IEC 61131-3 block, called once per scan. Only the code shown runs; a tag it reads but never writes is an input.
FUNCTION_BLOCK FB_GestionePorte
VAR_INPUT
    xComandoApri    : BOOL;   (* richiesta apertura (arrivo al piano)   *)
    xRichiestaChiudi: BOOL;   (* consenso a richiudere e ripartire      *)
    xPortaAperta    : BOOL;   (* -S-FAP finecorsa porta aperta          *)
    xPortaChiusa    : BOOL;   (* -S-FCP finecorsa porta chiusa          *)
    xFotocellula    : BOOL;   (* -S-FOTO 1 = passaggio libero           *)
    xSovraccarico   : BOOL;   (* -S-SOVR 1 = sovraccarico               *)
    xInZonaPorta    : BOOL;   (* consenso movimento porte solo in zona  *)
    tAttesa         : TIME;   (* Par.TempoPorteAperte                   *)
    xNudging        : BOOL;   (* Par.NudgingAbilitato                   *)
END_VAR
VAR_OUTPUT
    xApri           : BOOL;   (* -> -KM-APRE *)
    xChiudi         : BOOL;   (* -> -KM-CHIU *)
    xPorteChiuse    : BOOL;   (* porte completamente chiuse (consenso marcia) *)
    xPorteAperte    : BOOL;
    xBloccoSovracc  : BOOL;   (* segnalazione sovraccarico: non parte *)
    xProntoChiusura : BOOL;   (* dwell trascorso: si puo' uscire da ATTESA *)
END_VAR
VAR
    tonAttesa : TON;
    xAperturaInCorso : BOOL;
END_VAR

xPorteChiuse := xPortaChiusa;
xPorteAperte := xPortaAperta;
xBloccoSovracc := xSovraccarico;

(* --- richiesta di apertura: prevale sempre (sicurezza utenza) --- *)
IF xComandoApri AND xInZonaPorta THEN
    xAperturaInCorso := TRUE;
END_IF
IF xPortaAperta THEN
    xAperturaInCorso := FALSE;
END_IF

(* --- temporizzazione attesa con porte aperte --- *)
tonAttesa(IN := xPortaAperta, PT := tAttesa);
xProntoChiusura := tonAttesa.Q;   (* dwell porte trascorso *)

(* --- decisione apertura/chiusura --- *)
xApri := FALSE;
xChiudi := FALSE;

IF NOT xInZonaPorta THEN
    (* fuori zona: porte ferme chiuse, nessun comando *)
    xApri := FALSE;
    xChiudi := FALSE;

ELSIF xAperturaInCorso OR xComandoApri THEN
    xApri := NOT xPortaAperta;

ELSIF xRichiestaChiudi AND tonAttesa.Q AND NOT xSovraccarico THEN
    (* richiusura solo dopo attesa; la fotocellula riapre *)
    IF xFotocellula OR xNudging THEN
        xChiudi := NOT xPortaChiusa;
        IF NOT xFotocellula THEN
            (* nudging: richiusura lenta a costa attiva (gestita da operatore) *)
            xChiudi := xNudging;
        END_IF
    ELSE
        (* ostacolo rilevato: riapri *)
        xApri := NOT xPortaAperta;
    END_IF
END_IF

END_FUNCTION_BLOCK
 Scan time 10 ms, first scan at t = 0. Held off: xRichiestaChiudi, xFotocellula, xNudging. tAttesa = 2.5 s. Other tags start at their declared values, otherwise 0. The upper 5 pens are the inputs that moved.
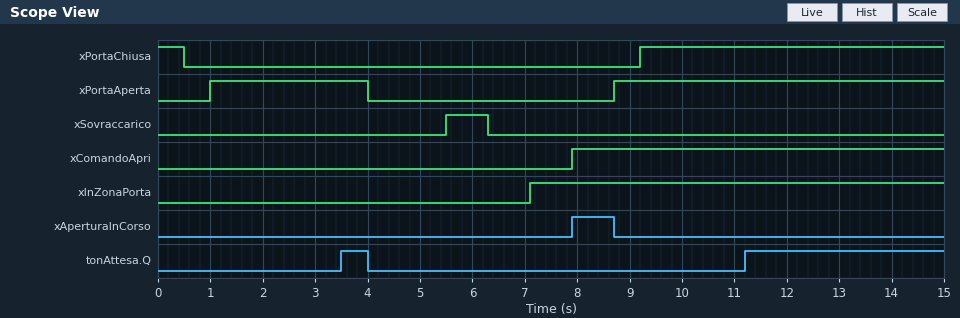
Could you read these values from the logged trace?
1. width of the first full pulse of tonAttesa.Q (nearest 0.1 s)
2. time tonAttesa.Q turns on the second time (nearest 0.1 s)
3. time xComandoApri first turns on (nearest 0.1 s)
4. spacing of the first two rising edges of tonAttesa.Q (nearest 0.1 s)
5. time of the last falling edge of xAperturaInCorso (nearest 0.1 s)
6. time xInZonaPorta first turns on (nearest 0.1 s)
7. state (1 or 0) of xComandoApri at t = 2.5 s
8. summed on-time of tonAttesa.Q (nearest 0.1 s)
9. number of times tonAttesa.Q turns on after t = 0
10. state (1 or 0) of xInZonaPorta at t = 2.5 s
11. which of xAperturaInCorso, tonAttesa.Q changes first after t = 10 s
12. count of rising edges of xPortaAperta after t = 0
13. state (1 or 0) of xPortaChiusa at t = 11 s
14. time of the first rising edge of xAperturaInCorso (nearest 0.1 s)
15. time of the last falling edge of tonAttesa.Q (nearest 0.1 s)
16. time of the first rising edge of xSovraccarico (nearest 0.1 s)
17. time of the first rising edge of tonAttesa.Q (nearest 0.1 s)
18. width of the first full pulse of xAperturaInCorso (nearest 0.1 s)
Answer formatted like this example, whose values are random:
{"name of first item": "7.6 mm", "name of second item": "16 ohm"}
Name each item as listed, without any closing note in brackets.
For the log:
{"width of the first full pulse of tonAttesa.Q": "0.5 s", "time tonAttesa.Q turns on the second time": "11.2 s", "time xComandoApri first turns on": "7.9 s", "spacing of the first two rising edges of tonAttesa.Q": "7.7 s", "time of the last falling edge of xAperturaInCorso": "8.7 s", "time xInZonaPorta first turns on": "7.1 s", "state (1 or 0) of xComandoApri at t = 2.5 s": "0", "summed on-time of tonAttesa.Q": "4.3 s", "number of times tonAttesa.Q turns on after t = 0": "2", "state (1 or 0) of xInZonaPorta at t = 2.5 s": "0", "which of xAperturaInCorso, tonAttesa.Q changes first after t = 10 s": "tonAttesa.Q", "count of rising edges of xPortaAperta after t = 0": "2", "state (1 or 0) of xPortaChiusa at t = 11 s": "1", "time of the first rising edge of xAperturaInCorso": "7.9 s", "time of the last falling edge of tonAttesa.Q": "4.0 s", "time of the first rising edge of xSovraccarico": "5.5 s", "time of the first rising edge of tonAttesa.Q": "3.5 s", "width of the first full pulse of xAperturaInCorso": "0.8 s"}
